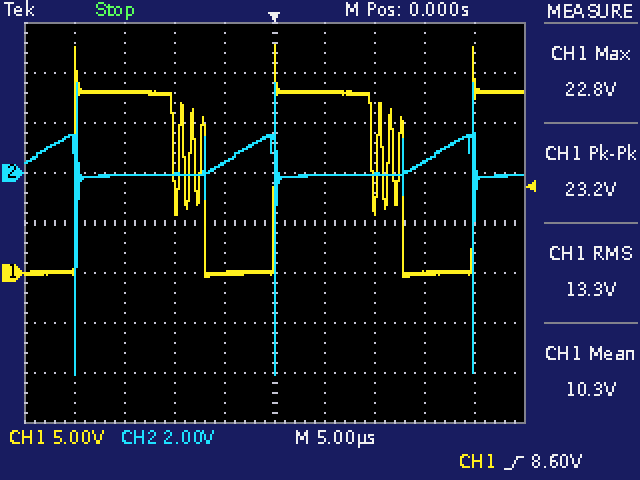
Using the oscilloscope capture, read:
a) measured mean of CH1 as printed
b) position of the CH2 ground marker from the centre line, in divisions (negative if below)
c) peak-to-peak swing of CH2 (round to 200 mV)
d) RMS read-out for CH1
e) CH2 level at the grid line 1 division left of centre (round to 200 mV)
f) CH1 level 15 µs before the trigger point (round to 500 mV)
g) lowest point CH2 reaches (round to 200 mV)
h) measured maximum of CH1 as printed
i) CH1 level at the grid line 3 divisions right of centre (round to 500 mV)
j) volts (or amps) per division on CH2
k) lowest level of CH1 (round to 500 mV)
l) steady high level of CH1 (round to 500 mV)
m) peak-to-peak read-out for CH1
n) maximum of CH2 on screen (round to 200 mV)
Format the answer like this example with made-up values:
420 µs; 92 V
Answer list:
10.3 V; +1.0 div; 11.6 V; 13.3 V; 400 mV; 18.0 V; -8.0 V; 22.8 V; 0.0 V; 2 V; -500 mV; 18.0 V; 23.2 V; 3.6 V
